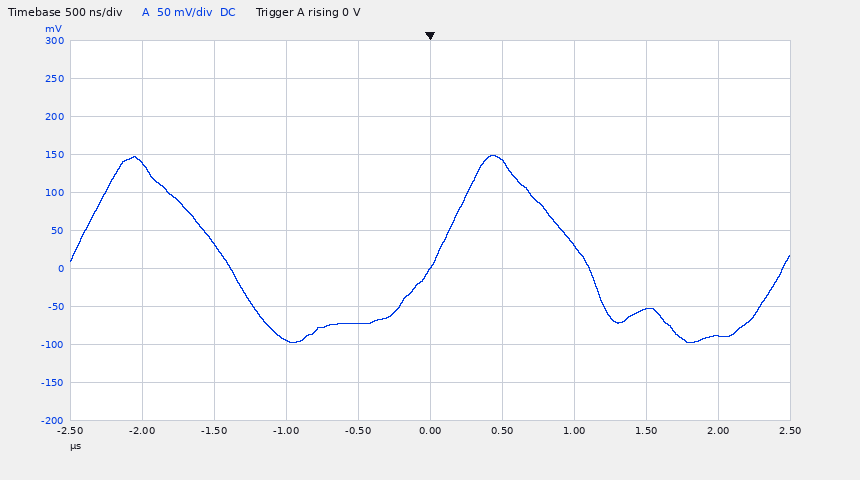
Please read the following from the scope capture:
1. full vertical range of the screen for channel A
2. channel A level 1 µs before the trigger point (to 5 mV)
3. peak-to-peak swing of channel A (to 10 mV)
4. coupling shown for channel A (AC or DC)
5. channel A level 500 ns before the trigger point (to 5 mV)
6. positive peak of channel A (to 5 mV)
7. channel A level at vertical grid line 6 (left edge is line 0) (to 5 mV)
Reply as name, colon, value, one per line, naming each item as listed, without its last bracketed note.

full vertical range of the screen for channel A: 500 mV
channel A level 1 µs before the trigger point: -95 mV
peak-to-peak swing of channel A: 250 mV
coupling shown for channel A: DC
channel A level 500 ns before the trigger point: -70 mV
positive peak of channel A: 150 mV
channel A level at vertical grid line 6 (left edge is line 0): 140 mV
